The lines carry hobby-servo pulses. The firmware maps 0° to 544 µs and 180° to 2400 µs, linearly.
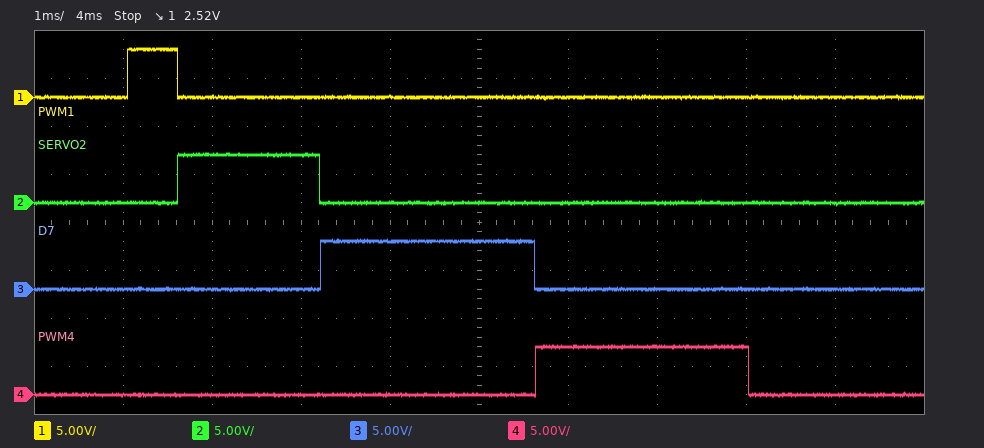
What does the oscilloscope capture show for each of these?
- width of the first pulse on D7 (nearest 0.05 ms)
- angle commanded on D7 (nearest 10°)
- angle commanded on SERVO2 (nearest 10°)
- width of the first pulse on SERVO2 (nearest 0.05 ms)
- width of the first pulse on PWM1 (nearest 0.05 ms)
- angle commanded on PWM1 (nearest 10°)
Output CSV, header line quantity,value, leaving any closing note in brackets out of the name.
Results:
quantity,value
width of the first pulse on D7,2.40 ms
angle commanded on D7,180°
angle commanded on SERVO2,100°
width of the first pulse on SERVO2,1.60 ms
width of the first pulse on PWM1,0.55 ms
angle commanded on PWM1,0°
